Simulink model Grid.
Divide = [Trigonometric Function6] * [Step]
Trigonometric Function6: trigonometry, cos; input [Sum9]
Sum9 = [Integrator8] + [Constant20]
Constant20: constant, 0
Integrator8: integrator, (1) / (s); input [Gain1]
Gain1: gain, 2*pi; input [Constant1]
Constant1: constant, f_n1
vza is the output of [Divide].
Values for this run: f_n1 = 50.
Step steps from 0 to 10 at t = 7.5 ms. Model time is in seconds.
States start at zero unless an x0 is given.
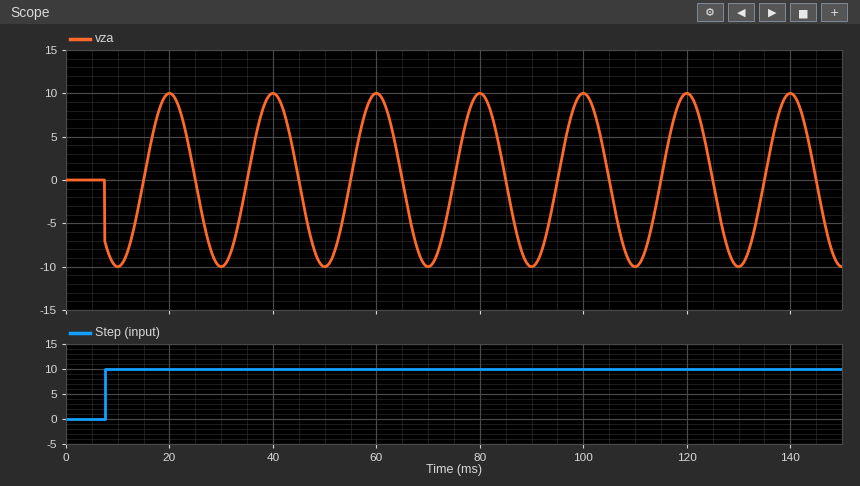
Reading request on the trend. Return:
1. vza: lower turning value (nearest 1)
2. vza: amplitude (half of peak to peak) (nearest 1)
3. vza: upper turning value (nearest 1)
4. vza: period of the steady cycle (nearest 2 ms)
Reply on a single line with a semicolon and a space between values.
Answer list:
-10; 10; 10; 20 ms
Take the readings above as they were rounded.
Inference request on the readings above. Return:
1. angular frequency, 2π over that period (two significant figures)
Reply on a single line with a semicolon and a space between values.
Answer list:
0.31 rad/ms
